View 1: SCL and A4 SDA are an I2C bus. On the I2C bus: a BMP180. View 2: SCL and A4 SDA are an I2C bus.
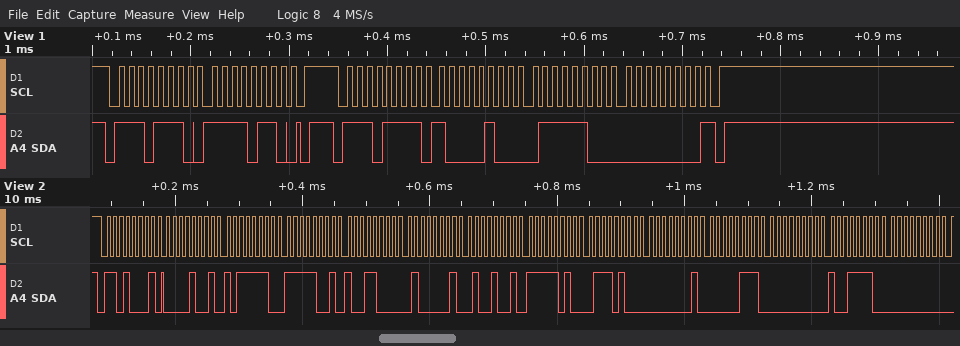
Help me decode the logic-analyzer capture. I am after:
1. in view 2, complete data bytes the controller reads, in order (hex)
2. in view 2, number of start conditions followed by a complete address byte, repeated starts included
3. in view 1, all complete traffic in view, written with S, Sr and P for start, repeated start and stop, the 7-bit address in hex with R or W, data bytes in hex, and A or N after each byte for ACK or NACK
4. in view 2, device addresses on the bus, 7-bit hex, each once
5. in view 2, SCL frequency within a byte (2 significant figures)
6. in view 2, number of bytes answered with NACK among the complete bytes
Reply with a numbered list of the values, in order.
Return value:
1. 09 BE F9 98 41 49 FA 74 01 07 00 9E 00
2. 1
3. S 77W A F6 A P S 77R A 84 A 7C A 00 N P
4. 0x68
5. 100 kHz
6. 0
